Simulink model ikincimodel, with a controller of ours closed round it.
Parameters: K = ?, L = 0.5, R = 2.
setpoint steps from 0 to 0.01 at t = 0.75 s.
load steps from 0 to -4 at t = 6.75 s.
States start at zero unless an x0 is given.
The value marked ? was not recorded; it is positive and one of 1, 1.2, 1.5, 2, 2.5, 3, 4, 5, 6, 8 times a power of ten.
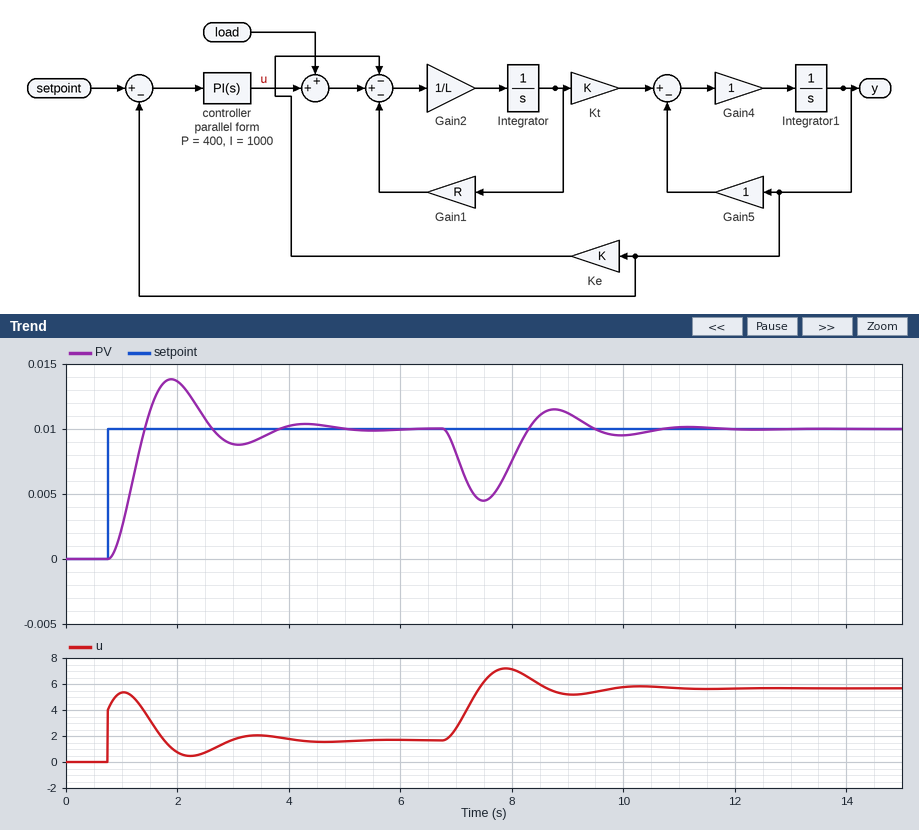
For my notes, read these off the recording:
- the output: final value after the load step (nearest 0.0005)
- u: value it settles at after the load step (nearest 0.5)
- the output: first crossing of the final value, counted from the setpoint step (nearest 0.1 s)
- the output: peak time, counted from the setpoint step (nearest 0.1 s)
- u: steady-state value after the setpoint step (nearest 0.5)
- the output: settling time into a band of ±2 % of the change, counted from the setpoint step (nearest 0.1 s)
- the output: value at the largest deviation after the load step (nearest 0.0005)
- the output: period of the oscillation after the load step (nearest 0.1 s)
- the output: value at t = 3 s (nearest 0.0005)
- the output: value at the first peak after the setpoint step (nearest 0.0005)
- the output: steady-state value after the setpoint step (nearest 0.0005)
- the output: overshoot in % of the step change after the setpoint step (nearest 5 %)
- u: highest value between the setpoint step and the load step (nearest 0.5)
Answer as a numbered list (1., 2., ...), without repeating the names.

1. 0.0100
2. 5.5
3. 0.7 s
4. 1.1 s
5. 1.5
6. 4.0 s
7. 0.0045
8. 2.5 s
9. 0.0090
10. 0.0140
11. 0.0100
12. 40 %
13. 5.5
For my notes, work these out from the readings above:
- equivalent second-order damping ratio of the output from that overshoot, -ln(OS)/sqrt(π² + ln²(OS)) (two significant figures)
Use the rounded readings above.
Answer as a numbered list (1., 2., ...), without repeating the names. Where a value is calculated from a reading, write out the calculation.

1. ln(0.4) = -0.916; 0.916 / sqrt(9.870 + 0.840) = 0.28
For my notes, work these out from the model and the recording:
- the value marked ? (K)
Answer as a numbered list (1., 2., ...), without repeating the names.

1. 0.012
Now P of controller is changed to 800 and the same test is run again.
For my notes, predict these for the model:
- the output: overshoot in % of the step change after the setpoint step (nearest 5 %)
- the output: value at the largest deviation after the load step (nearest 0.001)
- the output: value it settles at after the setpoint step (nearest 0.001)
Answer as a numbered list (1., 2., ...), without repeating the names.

1. 25 %
2. 0.006
3. 0.010
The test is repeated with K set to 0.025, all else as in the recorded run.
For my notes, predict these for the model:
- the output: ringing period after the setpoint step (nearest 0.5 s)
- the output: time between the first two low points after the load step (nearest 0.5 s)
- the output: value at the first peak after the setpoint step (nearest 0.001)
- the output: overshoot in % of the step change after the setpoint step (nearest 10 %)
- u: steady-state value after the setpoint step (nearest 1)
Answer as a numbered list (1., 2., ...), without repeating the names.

1. 1.5 s
2. 1.5 s
3. 0.015
4. 50 %
5. 1
